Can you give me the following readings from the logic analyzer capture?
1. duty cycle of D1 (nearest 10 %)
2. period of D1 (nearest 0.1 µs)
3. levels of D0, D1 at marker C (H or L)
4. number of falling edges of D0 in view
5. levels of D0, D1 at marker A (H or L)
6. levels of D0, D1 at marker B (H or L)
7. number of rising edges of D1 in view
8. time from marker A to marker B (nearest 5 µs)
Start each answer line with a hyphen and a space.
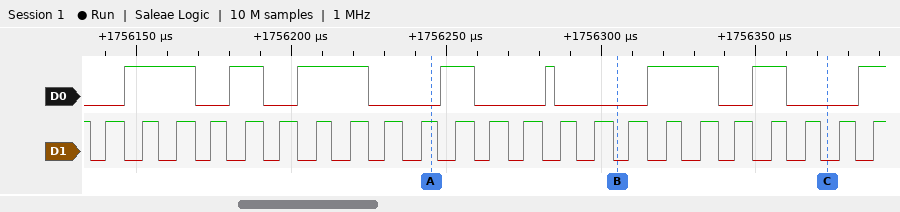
- 50 %
- 11.3 µs
- D0=L, D1=L
- 7
- D0=L, D1=H
- D0=L, D1=L
- 23
- 60 µs
